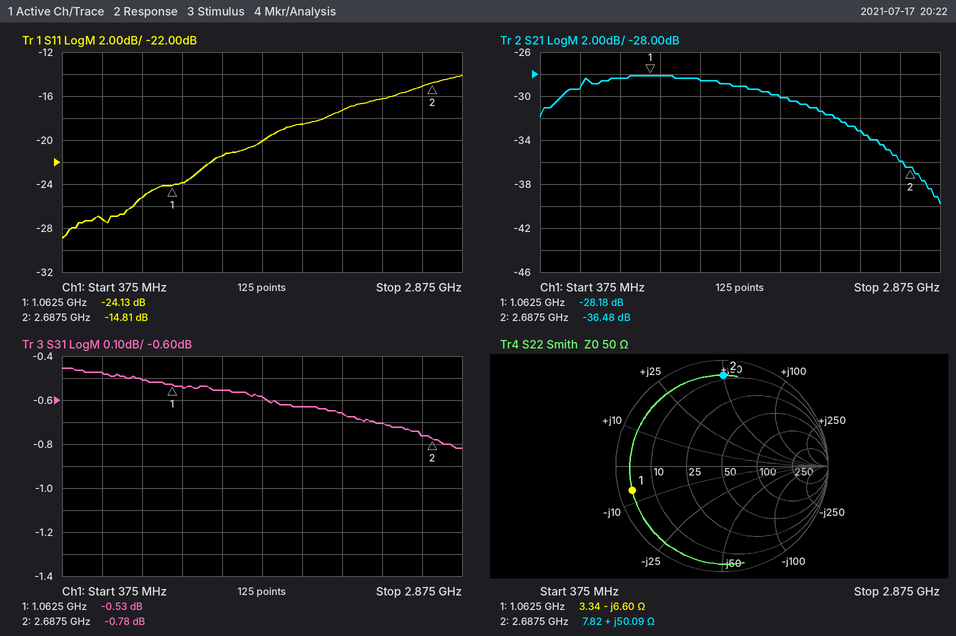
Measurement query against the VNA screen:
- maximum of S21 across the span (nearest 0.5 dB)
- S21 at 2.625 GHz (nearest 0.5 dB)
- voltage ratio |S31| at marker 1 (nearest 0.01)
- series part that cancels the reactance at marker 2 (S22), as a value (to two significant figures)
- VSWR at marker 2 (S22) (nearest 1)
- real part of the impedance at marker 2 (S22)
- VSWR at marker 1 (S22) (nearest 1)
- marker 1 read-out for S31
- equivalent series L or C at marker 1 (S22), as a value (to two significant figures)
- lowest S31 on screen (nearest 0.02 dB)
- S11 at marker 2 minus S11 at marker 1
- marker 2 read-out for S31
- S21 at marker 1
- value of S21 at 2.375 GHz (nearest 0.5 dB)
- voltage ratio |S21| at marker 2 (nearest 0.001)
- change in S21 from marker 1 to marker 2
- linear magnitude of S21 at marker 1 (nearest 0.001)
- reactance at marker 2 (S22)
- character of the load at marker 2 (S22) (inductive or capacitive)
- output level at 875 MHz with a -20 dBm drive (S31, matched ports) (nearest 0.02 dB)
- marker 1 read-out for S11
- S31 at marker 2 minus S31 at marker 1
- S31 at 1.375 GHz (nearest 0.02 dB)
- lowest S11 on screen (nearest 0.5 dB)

-28.0 dB
-36.0 dB
0.94
1.2 pF
13
7.82 Ω
15
-0.53 dB
23 pF
-0.82 dB
9.32 dB
-0.78 dB
-28.18 dB
-33.0 dB
0.015
-8.30 dB
0.039
+50.09 Ω
inductive
-20.50 dBm
-24.13 dB
-0.25 dB
-0.56 dB
-29.0 dB
